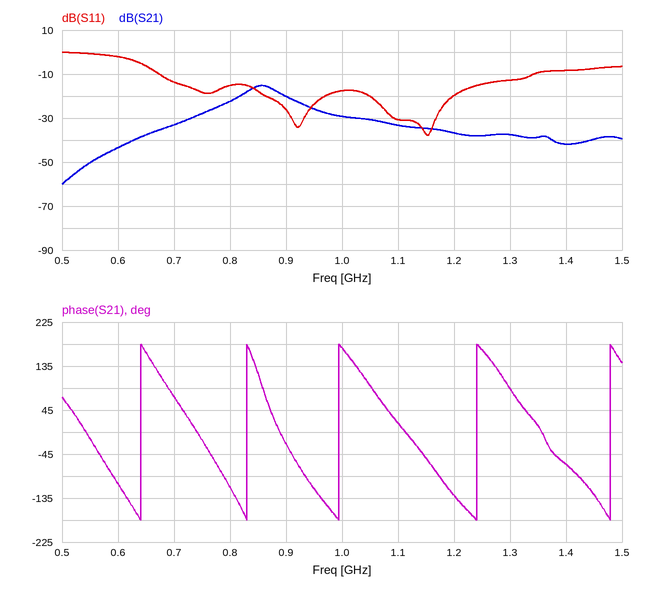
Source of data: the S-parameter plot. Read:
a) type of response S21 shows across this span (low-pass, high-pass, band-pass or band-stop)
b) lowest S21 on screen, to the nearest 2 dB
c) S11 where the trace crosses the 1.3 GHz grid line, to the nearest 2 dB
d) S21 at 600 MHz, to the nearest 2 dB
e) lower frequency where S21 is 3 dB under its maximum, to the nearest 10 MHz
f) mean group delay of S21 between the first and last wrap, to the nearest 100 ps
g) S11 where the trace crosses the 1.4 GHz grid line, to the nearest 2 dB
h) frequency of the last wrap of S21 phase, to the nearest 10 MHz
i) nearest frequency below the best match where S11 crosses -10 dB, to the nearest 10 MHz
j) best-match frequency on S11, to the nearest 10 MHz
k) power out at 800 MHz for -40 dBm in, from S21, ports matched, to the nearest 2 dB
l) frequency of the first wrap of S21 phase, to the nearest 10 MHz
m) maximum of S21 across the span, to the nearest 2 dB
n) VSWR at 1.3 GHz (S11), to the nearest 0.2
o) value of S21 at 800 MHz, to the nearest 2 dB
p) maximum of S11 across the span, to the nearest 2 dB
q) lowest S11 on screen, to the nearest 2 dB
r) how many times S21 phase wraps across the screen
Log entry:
band-pass
-60 dB
-12 dB
-44 dB
830 MHz
4.8 ns
-8 dB
1.48 GHz
670 MHz
1.15 GHz
-62 dBm
640 MHz
-16 dB
1.6
-22 dB
0 dB
-38 dB
5
